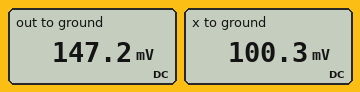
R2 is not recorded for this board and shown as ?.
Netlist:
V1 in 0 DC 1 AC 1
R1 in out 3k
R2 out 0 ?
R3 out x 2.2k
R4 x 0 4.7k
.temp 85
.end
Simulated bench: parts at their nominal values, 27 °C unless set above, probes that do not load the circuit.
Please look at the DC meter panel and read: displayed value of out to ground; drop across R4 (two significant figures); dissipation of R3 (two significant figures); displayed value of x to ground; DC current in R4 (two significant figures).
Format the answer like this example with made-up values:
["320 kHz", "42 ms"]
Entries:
["147.2 mV", "100 mV", "1.0 µW", "100.3 mV", "21 µA"]
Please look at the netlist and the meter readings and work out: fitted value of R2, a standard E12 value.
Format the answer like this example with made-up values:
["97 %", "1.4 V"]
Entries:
["560 Ω"]
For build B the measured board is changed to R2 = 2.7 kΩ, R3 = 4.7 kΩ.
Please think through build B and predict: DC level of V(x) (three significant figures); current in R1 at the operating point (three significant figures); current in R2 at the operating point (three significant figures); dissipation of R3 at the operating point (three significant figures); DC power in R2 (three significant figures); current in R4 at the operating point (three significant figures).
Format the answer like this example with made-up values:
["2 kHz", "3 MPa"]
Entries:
["206 mV", "196 µA", "152 µA", "9.01 µW", "62.7 µW", "43.8 µA"]
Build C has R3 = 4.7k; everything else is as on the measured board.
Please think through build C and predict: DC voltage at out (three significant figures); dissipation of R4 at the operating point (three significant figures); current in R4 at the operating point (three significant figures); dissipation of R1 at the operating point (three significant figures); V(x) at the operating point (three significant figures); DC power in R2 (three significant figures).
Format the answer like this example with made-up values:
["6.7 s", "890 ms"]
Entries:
["150 mV", "1.19 µW", "15.9 µA", "241 µW", "74.9 mV", "40.1 µW"]
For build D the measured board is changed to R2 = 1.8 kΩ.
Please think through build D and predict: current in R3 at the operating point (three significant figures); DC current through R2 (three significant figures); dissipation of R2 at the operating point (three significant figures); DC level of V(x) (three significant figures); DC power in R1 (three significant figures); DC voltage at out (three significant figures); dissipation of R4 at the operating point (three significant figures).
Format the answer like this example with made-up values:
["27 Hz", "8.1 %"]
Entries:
["46.7 µA", "179 µA", "57.8 µW", "220 mV", "153 µW", "322 mV", "10.3 µW"]
